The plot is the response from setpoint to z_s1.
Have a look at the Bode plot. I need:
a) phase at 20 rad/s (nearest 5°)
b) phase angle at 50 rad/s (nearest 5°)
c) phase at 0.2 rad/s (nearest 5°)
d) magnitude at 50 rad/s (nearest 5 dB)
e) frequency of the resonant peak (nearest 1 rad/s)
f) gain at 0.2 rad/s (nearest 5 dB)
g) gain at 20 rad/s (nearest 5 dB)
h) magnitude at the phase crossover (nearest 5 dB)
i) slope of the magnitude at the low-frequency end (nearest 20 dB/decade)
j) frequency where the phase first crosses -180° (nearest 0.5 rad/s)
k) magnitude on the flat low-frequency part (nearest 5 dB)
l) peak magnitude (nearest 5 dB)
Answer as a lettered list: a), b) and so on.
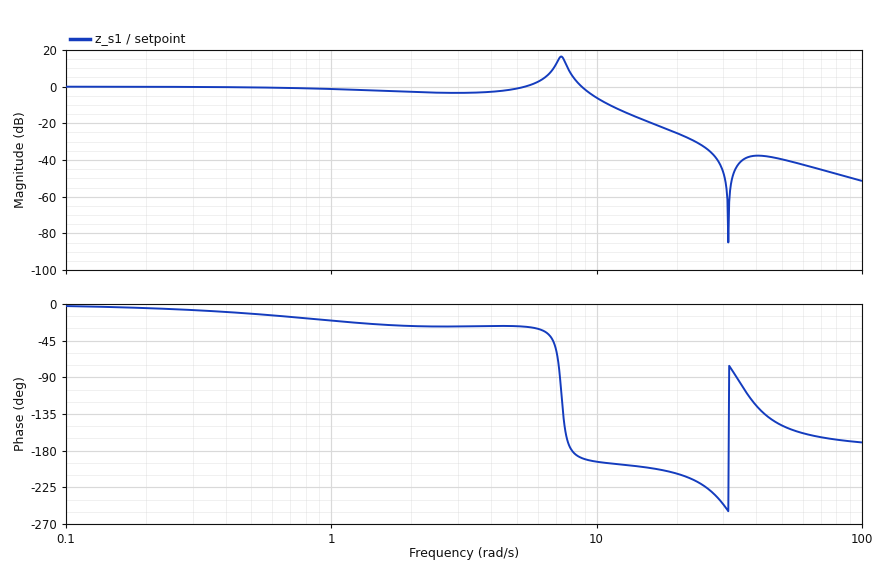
a) -210°
b) -150°
c) -5°
d) -40 dB
e) 7 rad/s
f) 0 dB
g) -25 dB
h) 5 dB
i) 0 dB/decade
j) 8.0 rad/s
k) 0 dB
l) 15 dB
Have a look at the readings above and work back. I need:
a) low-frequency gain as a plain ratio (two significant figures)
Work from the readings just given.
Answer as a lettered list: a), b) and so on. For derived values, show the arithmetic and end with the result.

a) 10^(0 / 20) = 1.0
